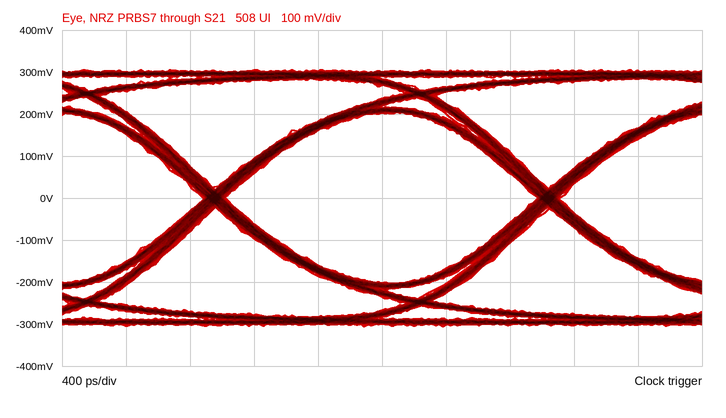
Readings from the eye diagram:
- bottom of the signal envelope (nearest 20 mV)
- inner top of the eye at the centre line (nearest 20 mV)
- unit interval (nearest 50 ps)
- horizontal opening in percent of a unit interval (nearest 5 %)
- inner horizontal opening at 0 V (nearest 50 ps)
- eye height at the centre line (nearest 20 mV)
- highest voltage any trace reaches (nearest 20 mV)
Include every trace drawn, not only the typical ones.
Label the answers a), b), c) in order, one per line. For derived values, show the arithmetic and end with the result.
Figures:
a) -300 mV
b) 200 mV
c) 2.10 ns
d) 1.95 ns / 2.10 ns ≈ 92.9 %, so 95 % to the nearest 5 %
e) 1.95 ns
f) 400 mV
g) 300 mV
